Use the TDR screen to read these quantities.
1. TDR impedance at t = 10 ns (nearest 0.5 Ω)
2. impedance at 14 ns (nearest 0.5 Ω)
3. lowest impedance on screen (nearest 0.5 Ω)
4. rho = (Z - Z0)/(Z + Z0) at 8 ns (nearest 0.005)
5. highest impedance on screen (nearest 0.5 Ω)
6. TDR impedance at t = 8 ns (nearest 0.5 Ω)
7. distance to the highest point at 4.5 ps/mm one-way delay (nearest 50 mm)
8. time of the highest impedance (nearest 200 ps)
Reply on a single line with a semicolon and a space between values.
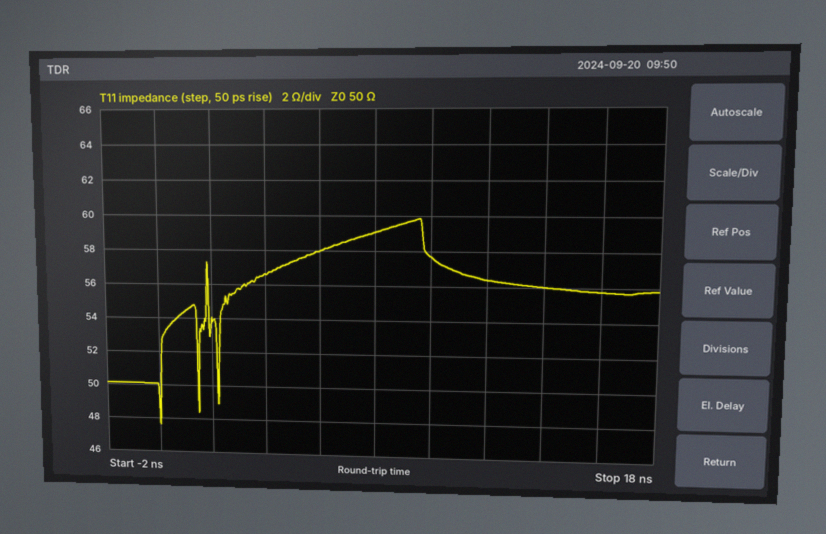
57.5 Ω; 56.0 Ω; 47.5 Ω; +0.085; 60.0 Ω; 59.0 Ω; 1.05 m; 9.6 ns
